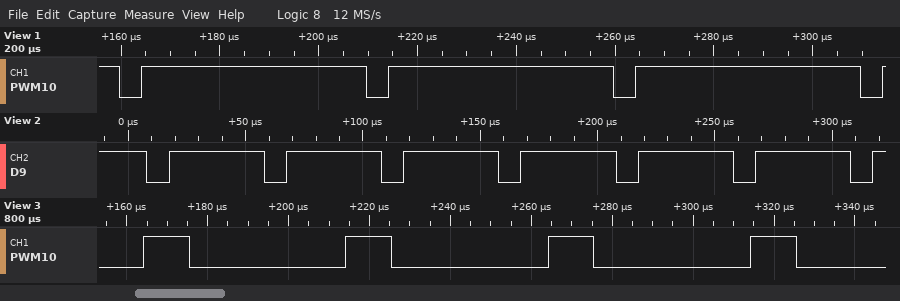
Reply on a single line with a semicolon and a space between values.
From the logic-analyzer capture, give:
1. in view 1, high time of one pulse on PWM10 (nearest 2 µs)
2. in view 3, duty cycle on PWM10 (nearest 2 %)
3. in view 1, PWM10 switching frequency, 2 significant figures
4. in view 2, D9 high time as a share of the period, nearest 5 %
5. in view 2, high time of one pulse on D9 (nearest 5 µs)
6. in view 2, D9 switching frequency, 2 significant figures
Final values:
46 µs; 22 %; 20 kHz; 80 %; 40 µs; 20 kHz
